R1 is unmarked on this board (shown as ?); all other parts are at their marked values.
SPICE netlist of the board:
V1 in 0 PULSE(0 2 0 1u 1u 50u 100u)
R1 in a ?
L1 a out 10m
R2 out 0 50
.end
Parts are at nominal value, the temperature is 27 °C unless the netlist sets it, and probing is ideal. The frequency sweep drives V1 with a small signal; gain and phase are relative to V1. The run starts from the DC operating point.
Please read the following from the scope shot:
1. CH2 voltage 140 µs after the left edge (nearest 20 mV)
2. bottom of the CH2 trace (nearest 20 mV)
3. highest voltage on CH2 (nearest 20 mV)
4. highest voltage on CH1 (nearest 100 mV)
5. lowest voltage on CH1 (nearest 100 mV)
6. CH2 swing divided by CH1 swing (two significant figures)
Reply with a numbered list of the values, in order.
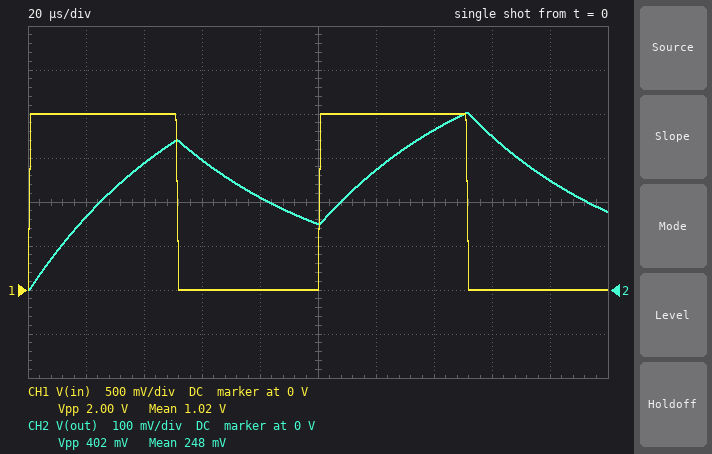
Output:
1. 360 mV
2. 0 V
3. 400 mV
4. 2.0 V
5. 0 V
6. 0.20
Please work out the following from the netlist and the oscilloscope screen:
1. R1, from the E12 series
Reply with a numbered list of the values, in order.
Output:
1. 120 Ω
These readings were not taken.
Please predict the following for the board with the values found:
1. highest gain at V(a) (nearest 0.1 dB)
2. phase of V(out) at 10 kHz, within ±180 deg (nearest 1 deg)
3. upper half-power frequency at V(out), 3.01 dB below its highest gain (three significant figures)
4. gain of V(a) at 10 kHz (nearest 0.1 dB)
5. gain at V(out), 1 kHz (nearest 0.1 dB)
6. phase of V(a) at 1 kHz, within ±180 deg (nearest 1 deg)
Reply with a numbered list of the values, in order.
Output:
1. 0 dB
2. -75 deg
3. 2.71 kHz
4. -0.3 dB
5. -11.2 dB
6. 31 deg
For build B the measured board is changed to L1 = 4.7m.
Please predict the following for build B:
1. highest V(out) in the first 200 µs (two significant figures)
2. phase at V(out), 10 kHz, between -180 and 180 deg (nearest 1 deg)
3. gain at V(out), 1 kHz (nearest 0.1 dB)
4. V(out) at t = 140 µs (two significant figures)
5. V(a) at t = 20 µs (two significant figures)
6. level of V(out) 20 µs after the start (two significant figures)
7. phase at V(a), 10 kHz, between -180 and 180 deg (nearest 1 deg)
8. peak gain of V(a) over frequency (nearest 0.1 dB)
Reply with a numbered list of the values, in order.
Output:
1. 510 mV
2. -60 deg
3. -10.8 dB
4. 470 mV
5. 1.3 V
6. 300 mV
7. 20 deg
8. 0 dB
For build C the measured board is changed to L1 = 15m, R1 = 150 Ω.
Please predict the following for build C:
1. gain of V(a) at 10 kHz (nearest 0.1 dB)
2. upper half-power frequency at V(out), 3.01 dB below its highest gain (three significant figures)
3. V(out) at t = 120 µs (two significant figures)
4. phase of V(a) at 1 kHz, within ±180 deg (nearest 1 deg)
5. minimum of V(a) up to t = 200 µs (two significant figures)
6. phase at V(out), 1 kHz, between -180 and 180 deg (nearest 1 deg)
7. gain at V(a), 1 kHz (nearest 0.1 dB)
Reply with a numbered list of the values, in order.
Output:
1. -0.2 dB
2. 2.12 kHz
3. 210 mV
4. 37 deg
5. -930 mV
6. -25 deg
7. -6.3 dB
